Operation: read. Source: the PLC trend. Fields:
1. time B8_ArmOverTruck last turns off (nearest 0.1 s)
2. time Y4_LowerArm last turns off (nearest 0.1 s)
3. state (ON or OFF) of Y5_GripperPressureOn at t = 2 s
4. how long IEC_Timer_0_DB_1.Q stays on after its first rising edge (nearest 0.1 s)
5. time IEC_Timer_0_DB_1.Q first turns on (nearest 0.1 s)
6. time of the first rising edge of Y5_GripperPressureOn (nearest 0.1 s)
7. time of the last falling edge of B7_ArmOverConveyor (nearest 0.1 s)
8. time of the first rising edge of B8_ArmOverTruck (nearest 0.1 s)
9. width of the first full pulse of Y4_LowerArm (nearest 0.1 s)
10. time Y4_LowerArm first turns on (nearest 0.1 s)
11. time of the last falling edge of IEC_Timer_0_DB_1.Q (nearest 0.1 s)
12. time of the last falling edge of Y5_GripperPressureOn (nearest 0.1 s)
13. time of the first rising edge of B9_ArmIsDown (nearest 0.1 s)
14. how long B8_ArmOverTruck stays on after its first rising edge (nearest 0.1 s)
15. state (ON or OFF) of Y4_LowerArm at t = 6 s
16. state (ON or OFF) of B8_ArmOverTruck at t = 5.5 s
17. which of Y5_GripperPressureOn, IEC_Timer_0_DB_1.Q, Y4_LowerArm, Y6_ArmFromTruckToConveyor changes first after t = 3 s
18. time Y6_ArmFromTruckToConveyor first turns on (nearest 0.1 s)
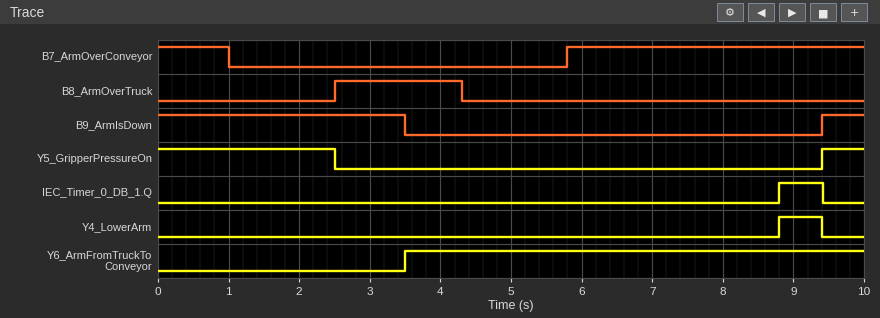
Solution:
4.3 s
9.4 s
ON
0.6 s
8.8 s
9.4 s
1.0 s
2.5 s
0.6 s
8.8 s
9.4 s
2.5 s
9.4 s
1.8 s
OFF
OFF
Y6_ArmFromTruckToConveyor
3.5 s
